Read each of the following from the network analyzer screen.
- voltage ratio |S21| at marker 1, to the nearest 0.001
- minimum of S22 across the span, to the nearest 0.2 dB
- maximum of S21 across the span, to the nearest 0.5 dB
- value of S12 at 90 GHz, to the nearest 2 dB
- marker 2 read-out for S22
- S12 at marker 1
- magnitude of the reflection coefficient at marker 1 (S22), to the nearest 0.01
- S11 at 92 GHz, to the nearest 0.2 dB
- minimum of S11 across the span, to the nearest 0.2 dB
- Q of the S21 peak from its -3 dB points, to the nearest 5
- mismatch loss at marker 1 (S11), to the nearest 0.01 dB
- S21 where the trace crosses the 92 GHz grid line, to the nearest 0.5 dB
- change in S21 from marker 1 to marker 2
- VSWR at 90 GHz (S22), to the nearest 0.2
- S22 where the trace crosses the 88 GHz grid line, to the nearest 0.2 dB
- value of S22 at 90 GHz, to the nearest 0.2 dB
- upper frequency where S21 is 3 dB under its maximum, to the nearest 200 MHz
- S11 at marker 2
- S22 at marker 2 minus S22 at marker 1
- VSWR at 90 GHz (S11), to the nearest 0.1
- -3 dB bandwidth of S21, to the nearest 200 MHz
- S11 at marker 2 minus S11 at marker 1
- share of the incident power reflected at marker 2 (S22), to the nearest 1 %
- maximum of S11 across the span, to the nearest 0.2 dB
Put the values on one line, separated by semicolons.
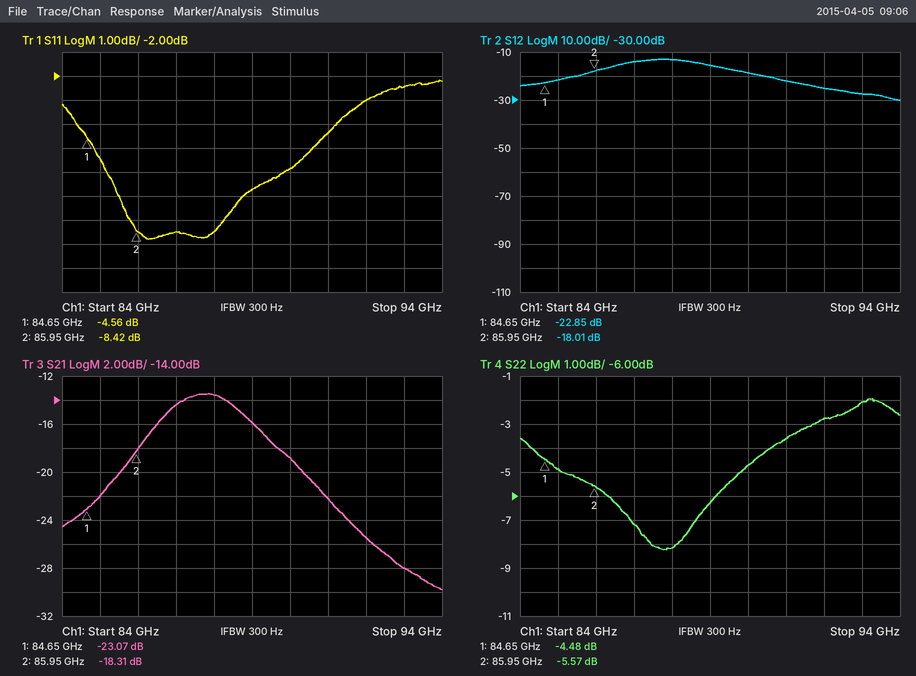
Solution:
0.070; -8.2 dB; -13.5 dB; -18 dB; -5.57 dB; -22.85 dB; 0.60; -3.0 dB; -8.8 dB; 30; 1.87 dB; -25.5 dB; 4.76 dB; 3.8; -8.2 dB; -4.8 dB; 89.2 GHz; -8.42 dB; -1.09 dB; 3.1; 2.8 GHz; -3.86 dB; 28 %; -2.2 dB
